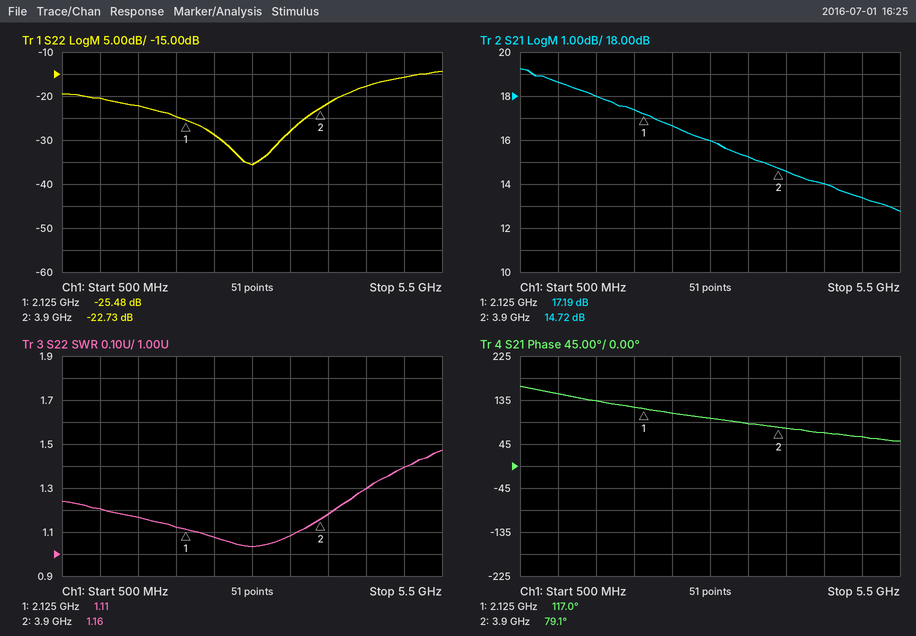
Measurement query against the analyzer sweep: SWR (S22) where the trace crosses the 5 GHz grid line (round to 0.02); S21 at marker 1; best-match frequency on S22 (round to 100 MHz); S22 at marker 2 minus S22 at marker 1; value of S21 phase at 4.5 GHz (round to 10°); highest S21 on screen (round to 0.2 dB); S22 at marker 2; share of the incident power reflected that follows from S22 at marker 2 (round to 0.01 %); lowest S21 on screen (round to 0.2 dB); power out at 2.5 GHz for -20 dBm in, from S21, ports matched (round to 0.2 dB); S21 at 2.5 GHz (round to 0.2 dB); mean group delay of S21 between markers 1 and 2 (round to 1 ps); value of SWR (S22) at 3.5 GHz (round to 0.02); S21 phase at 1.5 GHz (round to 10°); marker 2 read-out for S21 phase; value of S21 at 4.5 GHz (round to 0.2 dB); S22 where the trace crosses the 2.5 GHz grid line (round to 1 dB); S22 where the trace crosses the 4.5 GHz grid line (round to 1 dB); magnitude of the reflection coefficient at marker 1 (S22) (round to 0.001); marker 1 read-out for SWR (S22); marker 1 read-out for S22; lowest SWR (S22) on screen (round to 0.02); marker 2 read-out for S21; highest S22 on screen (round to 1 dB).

1.40
17.19 dB
3.0 GHz
2.75 dB
70°
19.2 dB
-22.73 dB
0.53 %
12.8 dB
-3.4 dBm
16.6 dB
59 ps
1.08
130°
79.1°
14.0 dB
-29 dB
-18 dB
0.053
1.11
-25.48 dB
1.04
14.72 dB
-14 dB
